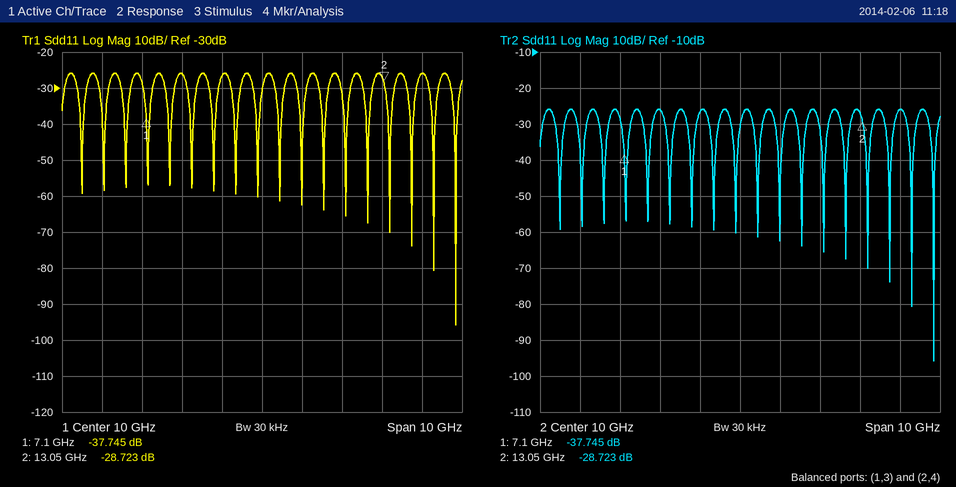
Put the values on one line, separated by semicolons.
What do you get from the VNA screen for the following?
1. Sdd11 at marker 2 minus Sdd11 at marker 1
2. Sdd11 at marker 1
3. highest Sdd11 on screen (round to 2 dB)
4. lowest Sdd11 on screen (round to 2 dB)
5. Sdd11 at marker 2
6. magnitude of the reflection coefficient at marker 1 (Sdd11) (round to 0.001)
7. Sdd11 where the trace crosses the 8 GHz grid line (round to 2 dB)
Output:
9.022 dB; -37.745 dB; -26 dB; -96 dB; -28.723 dB; 0.013; -26 dB
